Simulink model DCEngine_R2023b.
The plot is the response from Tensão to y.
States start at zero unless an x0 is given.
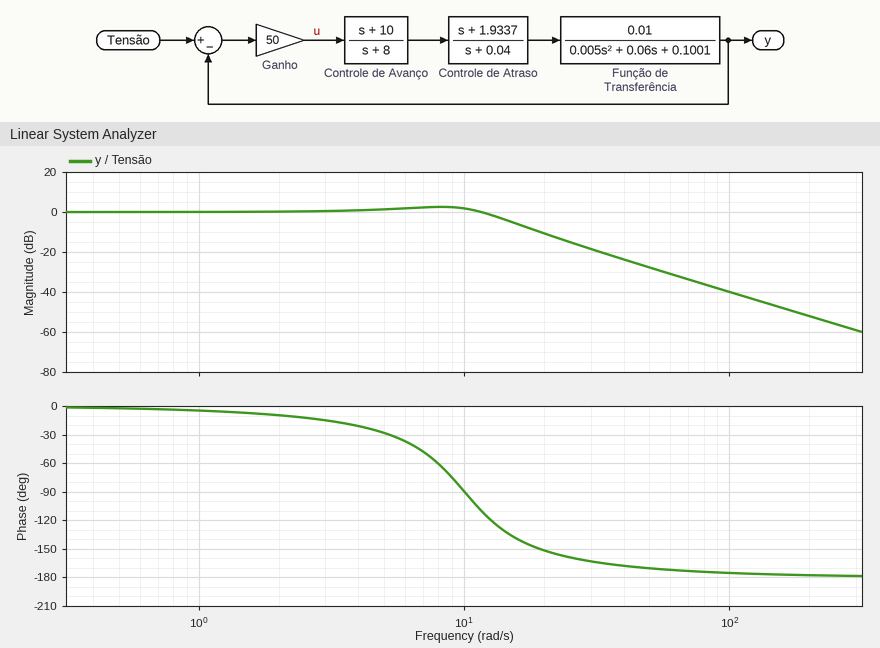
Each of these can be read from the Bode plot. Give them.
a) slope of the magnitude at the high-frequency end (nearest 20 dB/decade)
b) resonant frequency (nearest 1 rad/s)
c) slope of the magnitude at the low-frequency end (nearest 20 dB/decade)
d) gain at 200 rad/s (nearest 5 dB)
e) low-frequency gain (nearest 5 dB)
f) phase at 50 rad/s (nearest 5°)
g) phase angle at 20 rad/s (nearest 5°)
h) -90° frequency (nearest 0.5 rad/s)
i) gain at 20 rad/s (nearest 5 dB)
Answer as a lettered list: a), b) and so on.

a) -40 dB/decade
b) 8 rad/s
c) 0 dB/decade
d) -50 dB
e) 0 dB
f) -170°
g) -150°
h) 10.0 rad/s
i) -10 dB
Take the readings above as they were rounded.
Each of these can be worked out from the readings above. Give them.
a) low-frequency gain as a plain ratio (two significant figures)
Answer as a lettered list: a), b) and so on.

a) 1.0
